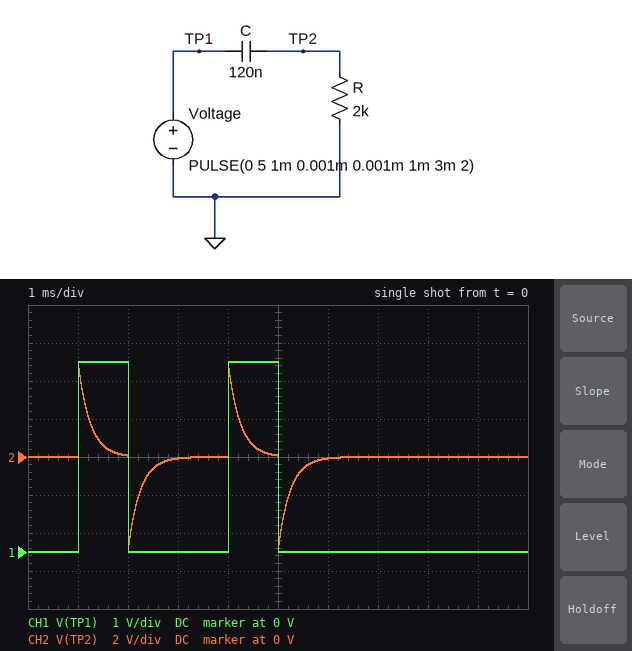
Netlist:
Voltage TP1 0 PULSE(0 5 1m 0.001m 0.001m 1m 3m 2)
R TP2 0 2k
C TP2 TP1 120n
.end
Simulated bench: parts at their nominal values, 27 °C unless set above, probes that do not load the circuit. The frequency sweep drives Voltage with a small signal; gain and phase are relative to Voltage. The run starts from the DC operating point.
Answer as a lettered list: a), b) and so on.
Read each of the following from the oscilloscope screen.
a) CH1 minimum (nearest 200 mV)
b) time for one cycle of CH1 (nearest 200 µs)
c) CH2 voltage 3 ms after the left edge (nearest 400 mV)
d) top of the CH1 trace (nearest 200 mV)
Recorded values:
a) 0 V
b) 3.0 ms
c) 0 V
d) 5.0 V
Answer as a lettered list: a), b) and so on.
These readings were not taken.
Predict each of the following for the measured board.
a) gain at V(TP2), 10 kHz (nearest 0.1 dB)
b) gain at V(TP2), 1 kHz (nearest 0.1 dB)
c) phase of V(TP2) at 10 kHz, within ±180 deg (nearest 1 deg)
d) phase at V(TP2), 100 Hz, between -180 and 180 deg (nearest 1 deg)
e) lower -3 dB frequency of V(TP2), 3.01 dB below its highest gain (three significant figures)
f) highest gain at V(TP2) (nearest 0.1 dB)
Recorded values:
a) 0 dB
b) -1.6 dB
c) 4 deg
d) 81 deg
e) 663 Hz
f) 0 dB
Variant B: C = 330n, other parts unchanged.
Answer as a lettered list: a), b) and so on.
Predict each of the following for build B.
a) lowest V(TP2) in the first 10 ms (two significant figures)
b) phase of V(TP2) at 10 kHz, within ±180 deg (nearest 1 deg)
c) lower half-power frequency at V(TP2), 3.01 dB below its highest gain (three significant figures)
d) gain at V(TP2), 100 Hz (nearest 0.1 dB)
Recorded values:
a) -3.9 V
b) 1 deg
c) 241 Hz
d) -8.3 dB
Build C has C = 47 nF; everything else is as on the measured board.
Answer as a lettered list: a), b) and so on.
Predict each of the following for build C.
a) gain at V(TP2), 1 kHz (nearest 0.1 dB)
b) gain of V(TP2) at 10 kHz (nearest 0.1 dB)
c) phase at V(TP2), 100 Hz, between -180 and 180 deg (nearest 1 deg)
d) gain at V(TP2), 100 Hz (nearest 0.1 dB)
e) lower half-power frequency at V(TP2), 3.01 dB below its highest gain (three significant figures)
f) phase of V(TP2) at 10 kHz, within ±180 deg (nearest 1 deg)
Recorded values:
a) -5.9 dB
b) -0.1 dB
c) 87 deg
d) -24.6 dB
e) 1.69 kHz
f) 10 deg
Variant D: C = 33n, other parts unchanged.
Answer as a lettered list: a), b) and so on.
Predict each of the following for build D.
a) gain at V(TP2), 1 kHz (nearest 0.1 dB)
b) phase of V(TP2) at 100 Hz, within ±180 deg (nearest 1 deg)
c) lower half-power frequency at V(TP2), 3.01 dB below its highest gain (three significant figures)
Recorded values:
a) -8.3 dB
b) 88 deg
c) 2.41 kHz
